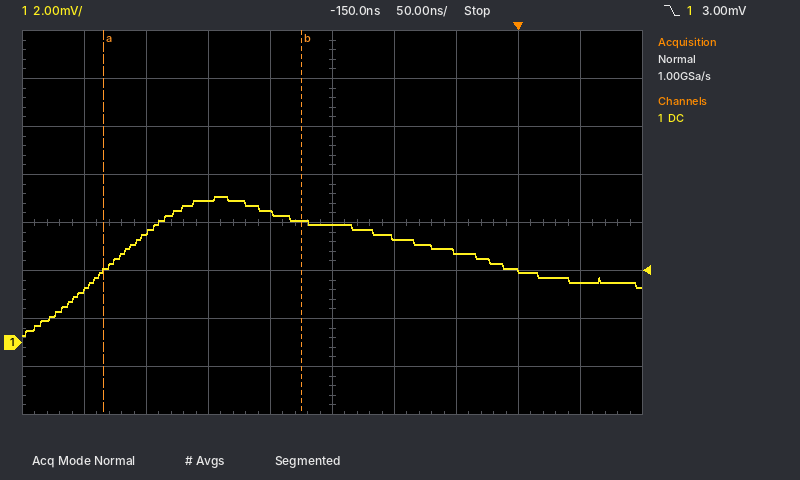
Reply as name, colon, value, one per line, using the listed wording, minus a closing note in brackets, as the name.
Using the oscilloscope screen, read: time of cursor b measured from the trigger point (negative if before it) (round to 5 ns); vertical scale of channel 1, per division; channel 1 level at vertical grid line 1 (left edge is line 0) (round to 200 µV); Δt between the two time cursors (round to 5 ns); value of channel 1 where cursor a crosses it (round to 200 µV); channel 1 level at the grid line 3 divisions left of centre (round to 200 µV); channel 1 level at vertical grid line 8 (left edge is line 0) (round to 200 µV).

time of cursor b measured from the trigger point (negative if before it): -175 ns
vertical scale of channel 1, per division: 2 mV
channel 1 level at vertical grid line 1 (left edge is line 0): 2.2 mV
Δt between the two time cursors: 160 ns
value of channel 1 where cursor a crosses it: 3.0 mV
channel 1 level at the grid line 3 divisions left of centre: 4.6 mV
channel 1 level at vertical grid line 8 (left edge is line 0): 3.0 mV
